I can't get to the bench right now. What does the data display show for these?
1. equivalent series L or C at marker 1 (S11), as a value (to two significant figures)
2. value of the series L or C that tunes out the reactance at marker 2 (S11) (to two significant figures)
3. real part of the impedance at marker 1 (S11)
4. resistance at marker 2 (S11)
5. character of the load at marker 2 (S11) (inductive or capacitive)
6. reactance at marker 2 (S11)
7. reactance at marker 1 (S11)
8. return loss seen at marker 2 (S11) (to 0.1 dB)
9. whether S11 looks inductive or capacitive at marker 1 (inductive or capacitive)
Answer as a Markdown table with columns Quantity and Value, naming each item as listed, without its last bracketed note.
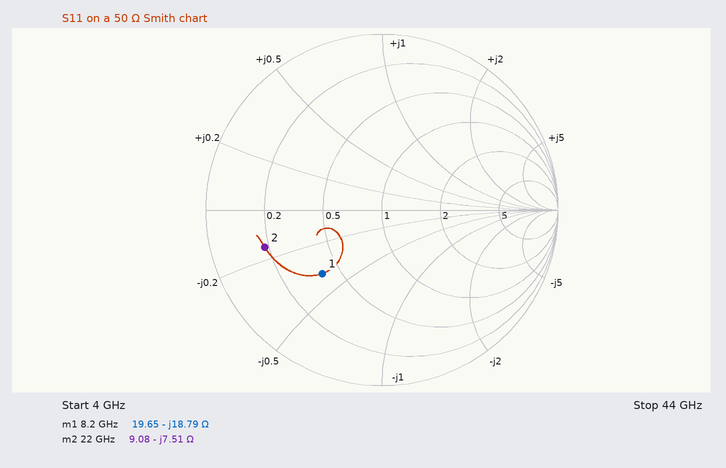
| Quantity | Value |
|---|---|
| equivalent series L or C at marker 1 (S11), as a value | 1.0 pF |
| value of the series L or C that tunes out the reactance at marker 2 (S11) | 54 pH |
| real part of the impedance at marker 1 | 19.65 Ω |
| resistance at marker 2 | 9.08 Ω |
| character of the load at marker 2 (S11) | capacitive |
| reactance at marker 2 | -7.51 Ω |
| reactance at marker 1 | -18.79 Ω |
| return loss seen at marker 2 (S11) | 3.1 dB |
| whether S11 looks inductive or capacitive at marker 1 | capacitive |
